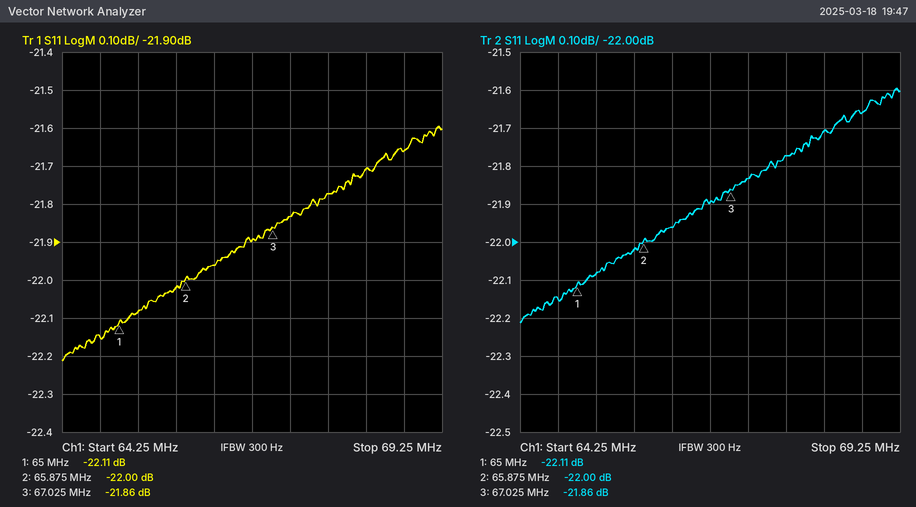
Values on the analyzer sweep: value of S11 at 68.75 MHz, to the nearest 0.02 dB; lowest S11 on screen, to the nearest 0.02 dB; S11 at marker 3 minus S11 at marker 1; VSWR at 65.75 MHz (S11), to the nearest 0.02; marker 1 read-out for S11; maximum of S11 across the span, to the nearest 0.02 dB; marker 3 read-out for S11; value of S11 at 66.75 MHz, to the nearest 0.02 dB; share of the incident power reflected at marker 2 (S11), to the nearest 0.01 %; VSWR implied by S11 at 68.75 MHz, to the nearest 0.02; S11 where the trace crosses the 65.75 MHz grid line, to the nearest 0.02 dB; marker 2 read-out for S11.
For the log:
-21.66 dB
-22.22 dB
0.25 dB
1.18
-22.11 dB
-21.60 dB
-21.86 dB
-21.90 dB
0.63 %
1.18
-22.02 dB
-22.00 dB
